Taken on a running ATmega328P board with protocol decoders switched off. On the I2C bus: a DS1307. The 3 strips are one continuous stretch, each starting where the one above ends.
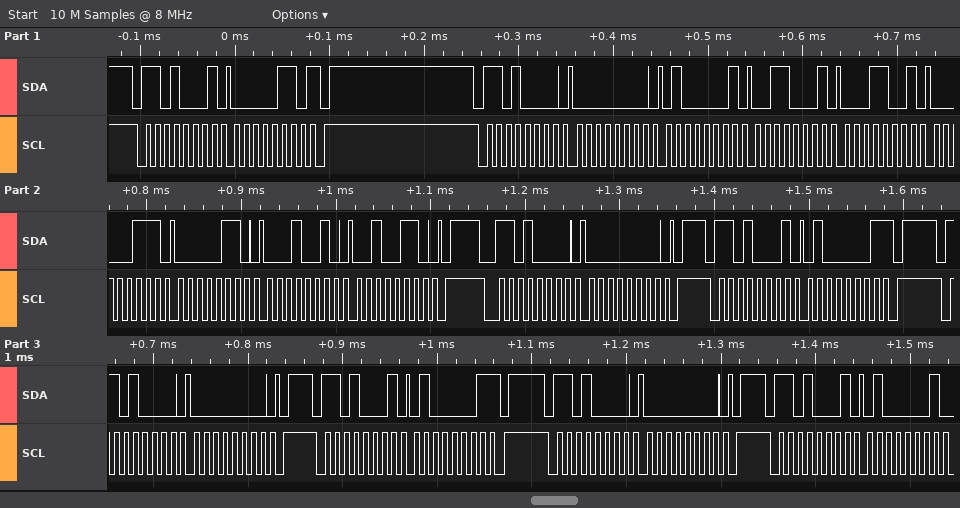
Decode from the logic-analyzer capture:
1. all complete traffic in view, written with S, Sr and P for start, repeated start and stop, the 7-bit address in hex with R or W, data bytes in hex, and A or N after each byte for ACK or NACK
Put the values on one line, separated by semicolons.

S 68R A 06 N P S 68W A 00 A 41 A 31 A 19 A 07 A 06 A 12 A 26 A P S 68W A 00 A P S 68R A 41 N P S 68W A 00 A P S 68R A 41 N P S 68W A 00 A P S 68R A 41 A
